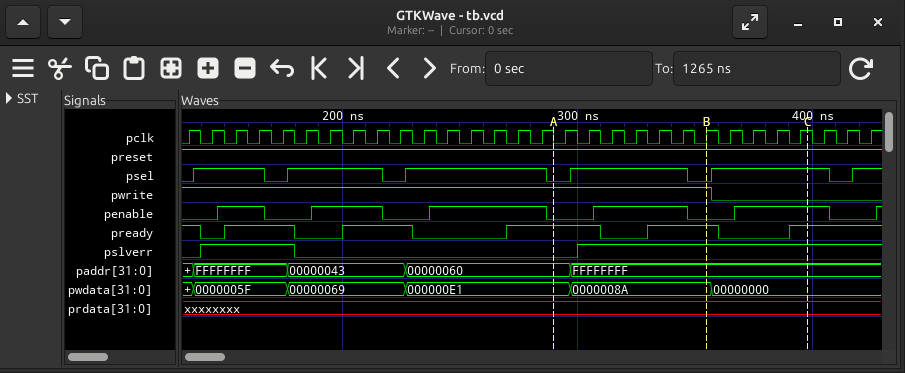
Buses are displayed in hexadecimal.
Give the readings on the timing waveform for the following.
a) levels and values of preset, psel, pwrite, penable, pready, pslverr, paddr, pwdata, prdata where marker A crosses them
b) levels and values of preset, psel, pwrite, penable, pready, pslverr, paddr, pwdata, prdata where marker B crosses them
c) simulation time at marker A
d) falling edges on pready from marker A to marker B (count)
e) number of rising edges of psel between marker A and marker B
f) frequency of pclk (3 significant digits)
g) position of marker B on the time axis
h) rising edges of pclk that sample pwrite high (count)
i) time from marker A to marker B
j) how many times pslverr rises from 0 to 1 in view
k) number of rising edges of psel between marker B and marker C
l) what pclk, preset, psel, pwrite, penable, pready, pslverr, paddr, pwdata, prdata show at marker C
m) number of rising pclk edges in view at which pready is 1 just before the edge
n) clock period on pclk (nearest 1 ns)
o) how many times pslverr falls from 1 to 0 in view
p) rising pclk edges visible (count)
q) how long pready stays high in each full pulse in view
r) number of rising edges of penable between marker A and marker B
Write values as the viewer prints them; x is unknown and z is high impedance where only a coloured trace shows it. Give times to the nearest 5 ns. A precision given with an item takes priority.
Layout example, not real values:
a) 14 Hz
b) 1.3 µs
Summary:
a) preset=1, psel=0, pwrite=1, penable=0, pready=1, pslverr=0, paddr=00000060, pwdata=000000E1, prdata=xxxxxxxx
b) preset=1, psel=0, pwrite=1, penable=0, pready=1, pslverr=1, paddr=FFFFFFFF, pwdata=0000008A, prdata=xxxxxxxx
c) 290 ns
d) 1
e) 1
f) 100 MHz
g) 355 ns
h) 23
i) 65 ns
j) 2
k) 1
l) pclk=1, preset=1, psel=1, pwrite=0, penable=1, pready=1, pslverr=1, paddr=FFFFFFFF, pwdata=00000000, prdata=xxxxxxxx
m) 18
n) 10 ns
o) 1
p) 30
q) 30 ns, 30 ns, 40 ns, 30 ns
r) 1
